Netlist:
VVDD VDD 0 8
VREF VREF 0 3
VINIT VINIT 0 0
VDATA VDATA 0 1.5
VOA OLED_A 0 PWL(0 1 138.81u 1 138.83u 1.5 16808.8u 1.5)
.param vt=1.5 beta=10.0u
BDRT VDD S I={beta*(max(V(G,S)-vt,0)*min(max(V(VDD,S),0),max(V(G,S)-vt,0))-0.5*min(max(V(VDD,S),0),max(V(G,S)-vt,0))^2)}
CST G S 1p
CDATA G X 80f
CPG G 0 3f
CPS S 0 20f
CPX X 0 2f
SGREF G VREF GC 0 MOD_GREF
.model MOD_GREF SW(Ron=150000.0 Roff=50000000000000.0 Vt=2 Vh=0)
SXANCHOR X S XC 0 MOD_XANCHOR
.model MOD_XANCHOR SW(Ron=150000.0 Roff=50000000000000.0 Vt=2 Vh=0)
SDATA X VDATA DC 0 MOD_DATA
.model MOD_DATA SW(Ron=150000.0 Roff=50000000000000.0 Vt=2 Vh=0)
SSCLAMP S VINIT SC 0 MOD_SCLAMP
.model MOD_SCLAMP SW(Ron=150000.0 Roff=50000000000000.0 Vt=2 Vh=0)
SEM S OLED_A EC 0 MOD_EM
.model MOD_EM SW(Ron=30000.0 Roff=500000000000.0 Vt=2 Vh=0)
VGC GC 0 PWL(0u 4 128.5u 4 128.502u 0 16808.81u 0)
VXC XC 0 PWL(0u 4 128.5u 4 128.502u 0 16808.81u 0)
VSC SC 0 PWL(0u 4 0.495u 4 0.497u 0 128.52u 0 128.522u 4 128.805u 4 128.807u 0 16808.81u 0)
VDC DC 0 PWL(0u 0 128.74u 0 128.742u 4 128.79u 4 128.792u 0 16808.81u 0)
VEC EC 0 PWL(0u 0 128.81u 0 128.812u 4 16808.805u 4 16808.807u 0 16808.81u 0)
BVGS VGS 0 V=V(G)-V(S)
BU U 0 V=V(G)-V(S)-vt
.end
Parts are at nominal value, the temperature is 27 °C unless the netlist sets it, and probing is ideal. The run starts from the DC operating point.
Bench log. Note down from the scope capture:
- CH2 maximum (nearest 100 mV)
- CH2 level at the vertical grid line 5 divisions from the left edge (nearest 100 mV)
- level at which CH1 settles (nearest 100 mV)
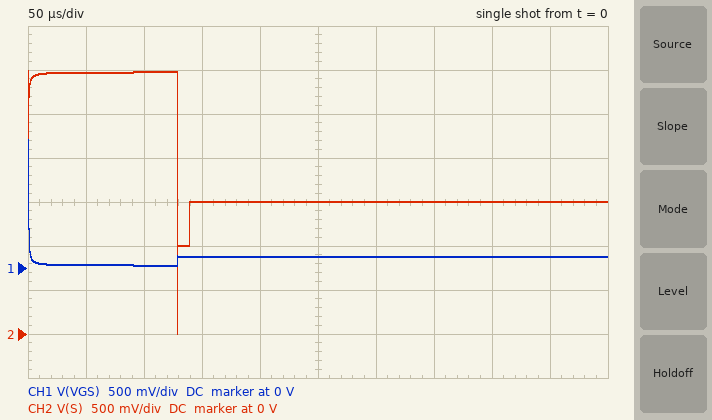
3.0 V
1.5 V
100 mV
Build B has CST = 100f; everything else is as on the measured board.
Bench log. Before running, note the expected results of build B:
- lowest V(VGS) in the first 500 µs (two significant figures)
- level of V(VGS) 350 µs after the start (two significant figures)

27 mV
550 mV
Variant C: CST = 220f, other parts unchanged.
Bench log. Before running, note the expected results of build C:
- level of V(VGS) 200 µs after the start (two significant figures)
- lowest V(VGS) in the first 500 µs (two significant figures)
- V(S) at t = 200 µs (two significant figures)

380 mV
27 mV
1.5 V
